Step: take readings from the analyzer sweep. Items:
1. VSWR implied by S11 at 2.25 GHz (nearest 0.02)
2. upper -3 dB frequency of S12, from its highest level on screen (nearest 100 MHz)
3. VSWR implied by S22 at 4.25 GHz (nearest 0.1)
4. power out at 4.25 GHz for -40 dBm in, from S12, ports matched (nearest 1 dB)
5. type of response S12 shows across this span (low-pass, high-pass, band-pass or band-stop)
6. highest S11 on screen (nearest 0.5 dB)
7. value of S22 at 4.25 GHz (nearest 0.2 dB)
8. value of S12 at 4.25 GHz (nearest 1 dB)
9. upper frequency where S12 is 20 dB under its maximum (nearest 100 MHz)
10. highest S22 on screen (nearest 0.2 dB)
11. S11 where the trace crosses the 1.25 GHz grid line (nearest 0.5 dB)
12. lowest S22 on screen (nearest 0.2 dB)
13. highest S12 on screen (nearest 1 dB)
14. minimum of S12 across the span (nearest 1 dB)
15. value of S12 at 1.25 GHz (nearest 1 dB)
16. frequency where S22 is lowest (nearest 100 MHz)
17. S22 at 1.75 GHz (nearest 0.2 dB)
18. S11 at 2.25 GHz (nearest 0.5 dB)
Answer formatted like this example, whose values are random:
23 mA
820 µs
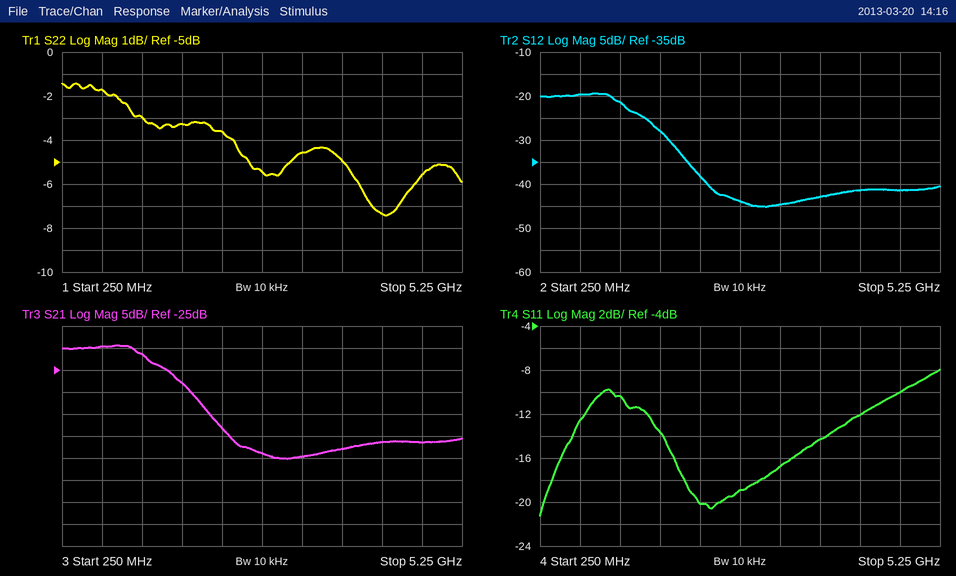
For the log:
1.22
1.3 GHz
2.5
-81 dBm
low-pass
-8.0 dB
-7.4 dB
-41 dB
2.3 GHz
-1.4 dB
-10.5 dB
-7.4 dB
-19 dB
-45 dB
-21 dB
4.3 GHz
-3.2 dB
-20.0 dB
